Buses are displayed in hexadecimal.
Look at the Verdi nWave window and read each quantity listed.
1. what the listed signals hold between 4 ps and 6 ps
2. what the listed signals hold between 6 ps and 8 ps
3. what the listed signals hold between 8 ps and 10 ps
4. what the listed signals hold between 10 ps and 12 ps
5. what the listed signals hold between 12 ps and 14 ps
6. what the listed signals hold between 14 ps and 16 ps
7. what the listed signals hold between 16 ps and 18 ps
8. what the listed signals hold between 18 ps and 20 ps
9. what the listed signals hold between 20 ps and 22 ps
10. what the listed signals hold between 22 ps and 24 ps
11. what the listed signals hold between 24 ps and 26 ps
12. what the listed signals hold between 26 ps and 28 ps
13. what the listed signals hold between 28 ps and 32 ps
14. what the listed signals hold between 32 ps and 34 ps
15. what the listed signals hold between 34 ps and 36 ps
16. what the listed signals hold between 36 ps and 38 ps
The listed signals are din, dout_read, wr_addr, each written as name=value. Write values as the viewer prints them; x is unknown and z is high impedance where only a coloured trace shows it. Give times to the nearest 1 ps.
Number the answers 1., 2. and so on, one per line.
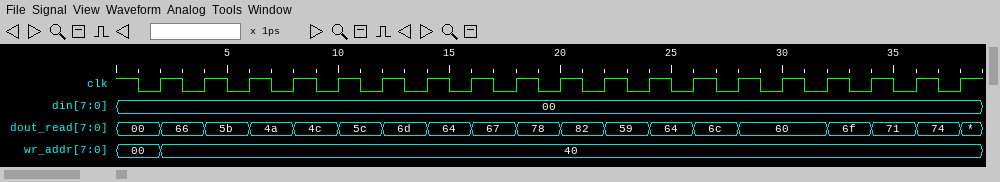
1. din=00, dout_read=5b, wr_addr=40
2. din=00, dout_read=4a, wr_addr=40
3. din=00, dout_read=4c, wr_addr=40
4. din=00, dout_read=5c, wr_addr=40
5. din=00, dout_read=6d, wr_addr=40
6. din=00, dout_read=64, wr_addr=40
7. din=00, dout_read=67, wr_addr=40
8. din=00, dout_read=78, wr_addr=40
9. din=00, dout_read=82, wr_addr=40
10. din=00, dout_read=59, wr_addr=40
11. din=00, dout_read=64, wr_addr=40
12. din=00, dout_read=6c, wr_addr=40
13. din=00, dout_read=60, wr_addr=40
14. din=00, dout_read=6f, wr_addr=40
15. din=00, dout_read=71, wr_addr=40
16. din=00, dout_read=74, wr_addr=40
